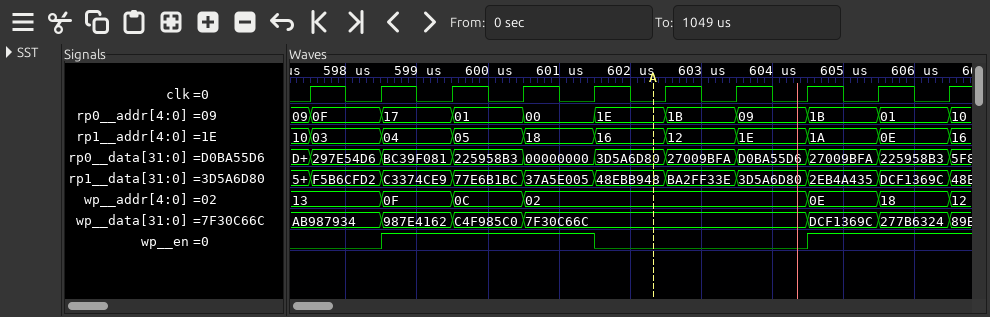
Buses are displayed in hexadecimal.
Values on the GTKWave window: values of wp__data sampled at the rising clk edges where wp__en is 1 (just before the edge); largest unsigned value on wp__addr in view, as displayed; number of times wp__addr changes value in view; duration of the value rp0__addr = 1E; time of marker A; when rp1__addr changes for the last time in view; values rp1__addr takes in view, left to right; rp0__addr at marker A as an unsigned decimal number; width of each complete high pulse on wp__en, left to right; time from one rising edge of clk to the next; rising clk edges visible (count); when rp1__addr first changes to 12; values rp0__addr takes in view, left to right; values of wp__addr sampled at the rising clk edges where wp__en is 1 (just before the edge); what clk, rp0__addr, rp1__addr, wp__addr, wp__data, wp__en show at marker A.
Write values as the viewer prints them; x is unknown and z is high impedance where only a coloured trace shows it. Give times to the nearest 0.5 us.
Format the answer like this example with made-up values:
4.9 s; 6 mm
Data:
987E4162, C4F985C0, 7F30C66C, DCF1369C, 277B6324; 18; 6; 1 us; 602.5 us; 606.5 us; 10, 03, 04, 05, 18, 16, 12, 1E, 1A, 0E, 16; 30; 3 us; 1 us; 10; 602.5 us; 09, 0F, 17, 01, 00, 1E, 1B, 09, 1B, 01, 10; 0F, 0C, 02, 0E, 18; clk=0, rp0__addr=1E, rp1__addr=16, wp__addr=02, wp__data=7F30C66C, wp__en=0
